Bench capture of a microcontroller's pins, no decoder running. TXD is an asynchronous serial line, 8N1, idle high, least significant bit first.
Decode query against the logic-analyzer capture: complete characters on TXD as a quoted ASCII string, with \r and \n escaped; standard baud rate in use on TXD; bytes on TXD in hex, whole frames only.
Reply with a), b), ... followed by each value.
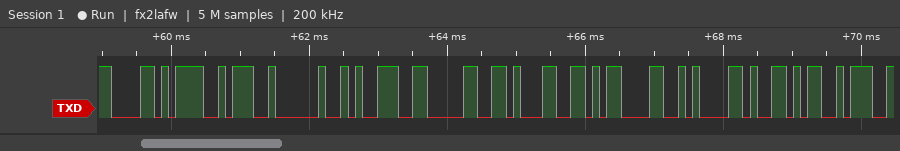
a) "X: 901\r\nY:"
b) 9600 baud
c) 0x58 0x3A 0x20 0x39 0x30 0x31 0x0D 0x0A 0x59 0x3A
